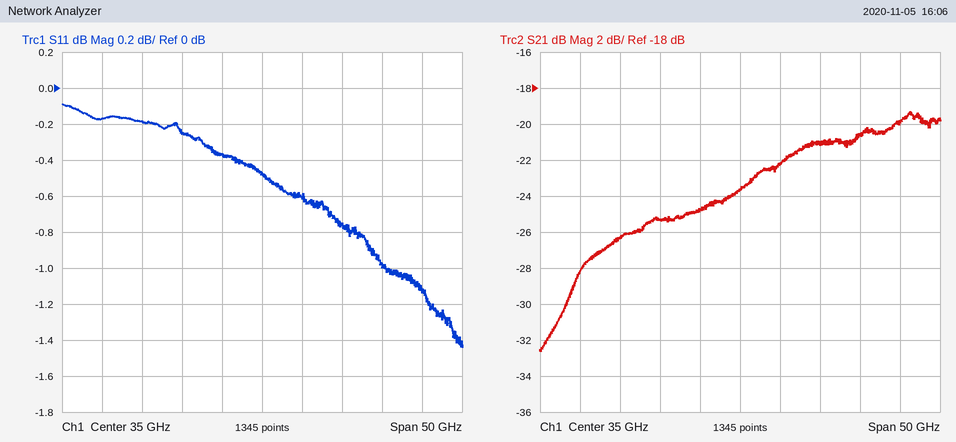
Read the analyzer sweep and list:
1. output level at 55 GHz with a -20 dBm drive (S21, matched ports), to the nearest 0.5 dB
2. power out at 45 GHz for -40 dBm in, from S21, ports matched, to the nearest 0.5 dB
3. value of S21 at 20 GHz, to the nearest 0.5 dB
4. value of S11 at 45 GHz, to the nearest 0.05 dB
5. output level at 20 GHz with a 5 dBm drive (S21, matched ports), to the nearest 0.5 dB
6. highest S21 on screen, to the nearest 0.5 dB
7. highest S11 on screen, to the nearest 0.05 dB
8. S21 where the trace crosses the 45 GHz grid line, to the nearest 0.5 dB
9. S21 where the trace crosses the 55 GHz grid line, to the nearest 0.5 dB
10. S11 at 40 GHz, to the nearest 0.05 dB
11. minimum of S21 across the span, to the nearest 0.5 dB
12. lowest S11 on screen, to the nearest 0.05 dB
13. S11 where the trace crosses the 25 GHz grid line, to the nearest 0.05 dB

-40.0 dBm
-61.0 dBm
-26.5 dB
-0.75 dB
-21.5 dBm
-19.5 dB
-0.10 dB
-21.0 dB
-20.0 dB
-0.60 dB
-32.5 dB
-1.45 dB
-0.25 dB
